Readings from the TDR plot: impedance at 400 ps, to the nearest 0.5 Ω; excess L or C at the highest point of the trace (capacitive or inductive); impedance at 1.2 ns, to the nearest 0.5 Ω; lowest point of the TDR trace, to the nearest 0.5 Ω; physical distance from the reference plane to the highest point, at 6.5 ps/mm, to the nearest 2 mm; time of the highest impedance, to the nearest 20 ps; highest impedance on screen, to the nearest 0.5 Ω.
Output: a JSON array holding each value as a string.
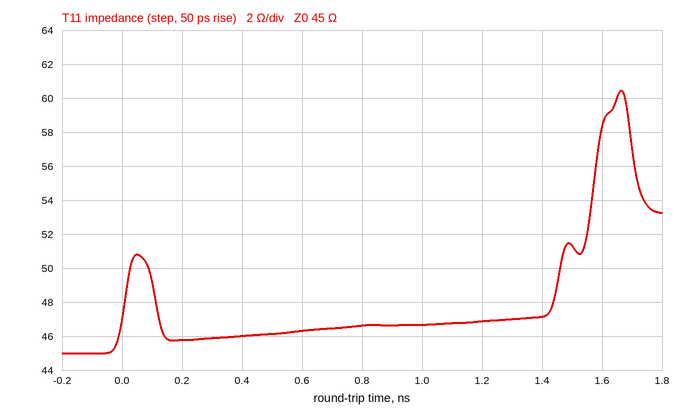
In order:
["46.0 Ω", "inductive", "47.0 Ω", "45.0 Ω", "128 mm", "1.66 ns", "60.5 Ω"]
